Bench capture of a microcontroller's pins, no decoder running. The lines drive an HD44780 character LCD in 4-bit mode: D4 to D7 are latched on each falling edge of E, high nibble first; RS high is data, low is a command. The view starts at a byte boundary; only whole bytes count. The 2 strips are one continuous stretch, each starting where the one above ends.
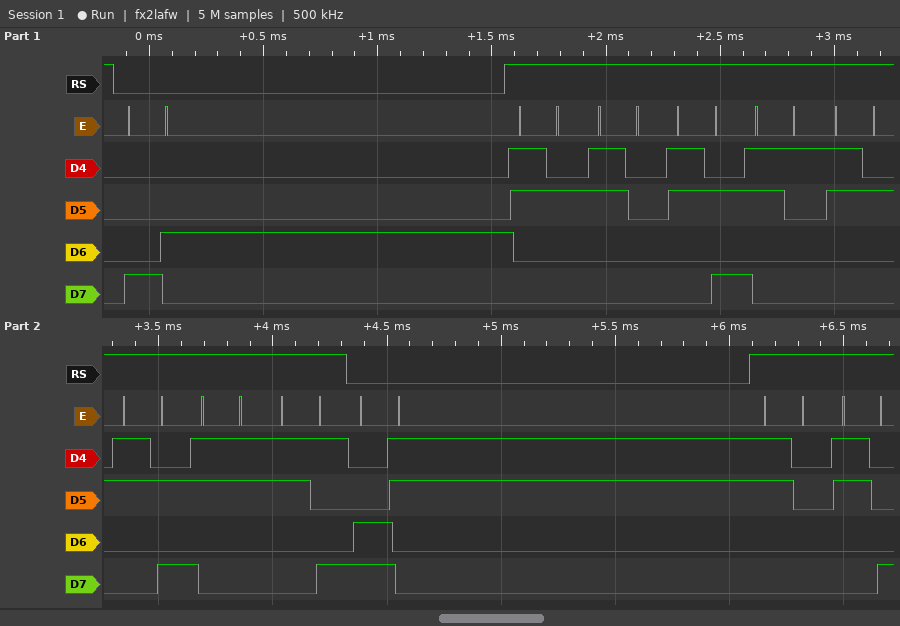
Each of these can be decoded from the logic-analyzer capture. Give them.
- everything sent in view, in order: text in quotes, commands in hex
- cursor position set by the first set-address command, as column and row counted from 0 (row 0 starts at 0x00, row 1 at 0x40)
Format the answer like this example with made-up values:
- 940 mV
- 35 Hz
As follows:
- 0x84 "20:12:39" 0xC3 "08"
- column 4, row 0
